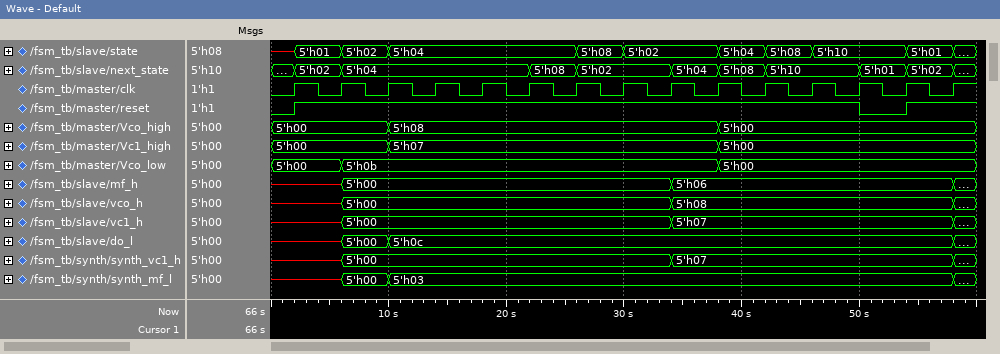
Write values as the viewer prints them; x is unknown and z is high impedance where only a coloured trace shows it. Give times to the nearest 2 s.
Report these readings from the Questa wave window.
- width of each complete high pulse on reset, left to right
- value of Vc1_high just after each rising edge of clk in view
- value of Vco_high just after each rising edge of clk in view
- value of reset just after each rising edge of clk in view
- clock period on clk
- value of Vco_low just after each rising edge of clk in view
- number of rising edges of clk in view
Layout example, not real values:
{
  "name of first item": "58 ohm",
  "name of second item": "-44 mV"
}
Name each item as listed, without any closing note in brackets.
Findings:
{
  "width of each complete high pulse on reset, left to right": "48 s",
  "value of Vc1_high just after each rising edge of clk in view": "5'h00, 5'h00, 5'h07, 5'h07, 5'h07, 5'h07, 5'h07, 5'h07, 5'h07, 5'h00, 5'h00, 5'h00, 5'h00, 5'h00, 5'h00",
  "value of Vco_high just after each rising edge of clk in view": "5'h00, 5'h00, 5'h08, 5'h08, 5'h08, 5'h08, 5'h08, 5'h08, 5'h08, 5'h00, 5'h00, 5'h00, 5'h00, 5'h00, 5'h00",
  "value of reset just after each rising edge of clk in view": "1 1 1 1 1 1 1 1 1 1 1 1 0 1 1",
  "clock period on clk": "4 s",
  "value of Vco_low just after each rising edge of clk in view": "5'h00, 5'h0b, 5'h0b, 5'h0b, 5'h0b, 5'h0b, 5'h0b, 5'h0b, 5'h0b, 5'h00, 5'h00, 5'h00, 5'h00, 5'h00, 5'h00",
  "number of rising edges of clk in view": "15"
}
